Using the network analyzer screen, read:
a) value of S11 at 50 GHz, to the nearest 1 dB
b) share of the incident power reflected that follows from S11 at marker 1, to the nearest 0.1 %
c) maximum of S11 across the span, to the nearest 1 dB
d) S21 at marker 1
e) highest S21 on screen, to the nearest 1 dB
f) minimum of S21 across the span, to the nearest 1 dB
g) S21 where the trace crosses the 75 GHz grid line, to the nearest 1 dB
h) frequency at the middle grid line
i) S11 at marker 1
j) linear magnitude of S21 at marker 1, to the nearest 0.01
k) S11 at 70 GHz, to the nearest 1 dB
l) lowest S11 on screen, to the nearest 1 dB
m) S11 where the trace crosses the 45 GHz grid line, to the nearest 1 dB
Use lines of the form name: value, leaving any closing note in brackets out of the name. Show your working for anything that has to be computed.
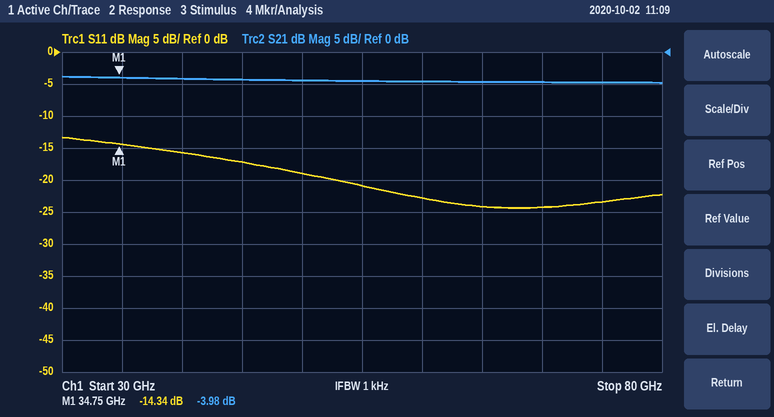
value of S11 at 50 GHz, to the nearest 1 dB: -19 dB
share of the incident power reflected that follows from S11 at marker 1, to the nearest 0.1 %: 10^(-14.34/10) ≈ 3.7 %
maximum of S11 across the span, to the nearest 1 dB: -13 dB
S21 at marker 1: -3.98 dB
highest S21 on screen, to the nearest 1 dB: -4 dB
minimum of S21 across the span, to the nearest 1 dB: -5 dB
S21 where the trace crosses the 75 GHz grid line, to the nearest 1 dB: -5 dB
frequency at the middle grid line: 55 GHz
S11 at marker 1: -14.34 dB
linear magnitude of S21 at marker 1, to the nearest 0.01: 10^(-3.98/20) ≈ 0.63
S11 at 70 GHz, to the nearest 1 dB: -24 dB
lowest S11 on screen, to the nearest 1 dB: -24 dB
S11 where the trace crosses the 45 GHz grid line, to the nearest 1 dB: -17 dB
